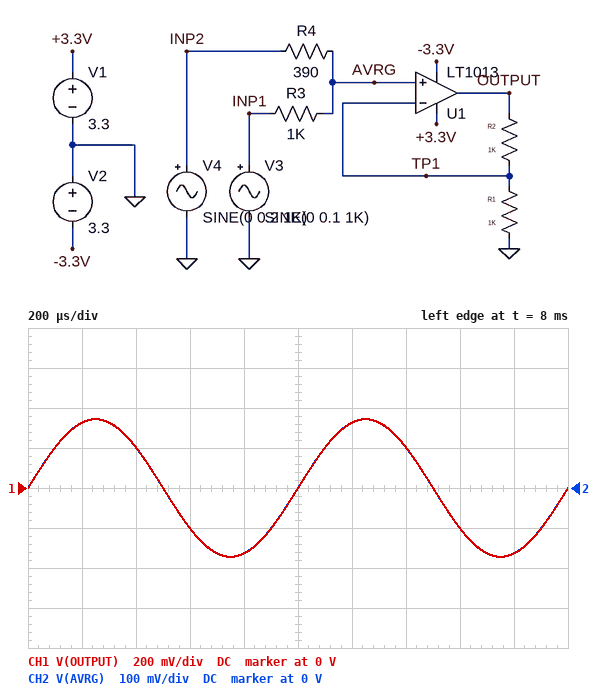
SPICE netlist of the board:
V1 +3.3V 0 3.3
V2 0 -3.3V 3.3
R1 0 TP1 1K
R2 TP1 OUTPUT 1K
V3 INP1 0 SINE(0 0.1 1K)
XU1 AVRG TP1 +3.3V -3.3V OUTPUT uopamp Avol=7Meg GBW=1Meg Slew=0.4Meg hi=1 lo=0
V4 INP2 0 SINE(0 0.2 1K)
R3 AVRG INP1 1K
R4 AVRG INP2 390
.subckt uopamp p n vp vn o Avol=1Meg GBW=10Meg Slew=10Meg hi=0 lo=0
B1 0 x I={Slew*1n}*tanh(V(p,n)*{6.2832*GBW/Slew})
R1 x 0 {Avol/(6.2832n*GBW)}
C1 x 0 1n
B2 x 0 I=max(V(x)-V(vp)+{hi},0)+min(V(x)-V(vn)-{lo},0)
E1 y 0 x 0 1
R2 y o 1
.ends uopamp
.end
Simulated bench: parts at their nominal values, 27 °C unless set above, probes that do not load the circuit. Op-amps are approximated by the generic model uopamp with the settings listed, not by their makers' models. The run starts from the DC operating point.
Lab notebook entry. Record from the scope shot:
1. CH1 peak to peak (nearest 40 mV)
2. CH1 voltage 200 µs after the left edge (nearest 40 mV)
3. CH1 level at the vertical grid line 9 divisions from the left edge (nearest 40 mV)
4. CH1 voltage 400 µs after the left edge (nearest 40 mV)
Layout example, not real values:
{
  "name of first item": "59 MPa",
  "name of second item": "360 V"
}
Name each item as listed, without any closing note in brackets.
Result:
{
  "CH1 peak to peak": "680 mV",
  "CH1 voltage 200 µs after the left edge": "320 mV",
  "CH1 level at the vertical grid line 9 divisions from the left edge": "-320 mV",
  "CH1 voltage 400 µs after the left edge": "200 mV"
}
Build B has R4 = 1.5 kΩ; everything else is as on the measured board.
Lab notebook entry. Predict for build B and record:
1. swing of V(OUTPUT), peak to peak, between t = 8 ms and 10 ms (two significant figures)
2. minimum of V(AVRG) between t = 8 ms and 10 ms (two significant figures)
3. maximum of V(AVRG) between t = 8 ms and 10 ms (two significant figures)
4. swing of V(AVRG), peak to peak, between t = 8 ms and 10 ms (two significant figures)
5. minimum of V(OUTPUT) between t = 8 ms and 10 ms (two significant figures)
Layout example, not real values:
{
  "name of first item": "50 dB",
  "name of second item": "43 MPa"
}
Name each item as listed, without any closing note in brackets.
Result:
{
  "swing of V(OUTPUT), peak to peak, between t = 8 ms and 10 ms": "560 mV",
  "minimum of V(AVRG) between t = 8 ms and 10 ms": "-140 mV",
  "maximum of V(AVRG) between t = 8 ms and 10 ms": "140 mV",
  "swing of V(AVRG), peak to peak, between t = 8 ms and 10 ms": "280 mV",
  "minimum of V(OUTPUT) between t = 8 ms and 10 ms": "-280 mV"
}
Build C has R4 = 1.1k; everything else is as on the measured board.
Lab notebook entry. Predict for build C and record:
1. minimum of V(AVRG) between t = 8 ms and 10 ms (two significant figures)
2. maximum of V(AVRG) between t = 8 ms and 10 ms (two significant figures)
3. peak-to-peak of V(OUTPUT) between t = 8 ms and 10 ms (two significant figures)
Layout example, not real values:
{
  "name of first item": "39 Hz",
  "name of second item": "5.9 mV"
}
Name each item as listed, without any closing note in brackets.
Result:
{
  "minimum of V(AVRG) between t = 8 ms and 10 ms": "-150 mV",
  "maximum of V(AVRG) between t = 8 ms and 10 ms": "150 mV",
  "peak-to-peak of V(OUTPUT) between t = 8 ms and 10 ms": "590 mV"
}
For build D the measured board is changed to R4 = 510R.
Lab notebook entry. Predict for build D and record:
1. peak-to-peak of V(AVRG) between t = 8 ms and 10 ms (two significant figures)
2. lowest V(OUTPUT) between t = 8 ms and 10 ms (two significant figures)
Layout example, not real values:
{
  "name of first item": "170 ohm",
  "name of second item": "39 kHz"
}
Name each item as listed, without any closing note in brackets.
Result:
{
  "peak-to-peak of V(AVRG) between t = 8 ms and 10 ms": "330 mV",
  "lowest V(OUTPUT) between t = 8 ms and 10 ms": "-330 mV"
}
